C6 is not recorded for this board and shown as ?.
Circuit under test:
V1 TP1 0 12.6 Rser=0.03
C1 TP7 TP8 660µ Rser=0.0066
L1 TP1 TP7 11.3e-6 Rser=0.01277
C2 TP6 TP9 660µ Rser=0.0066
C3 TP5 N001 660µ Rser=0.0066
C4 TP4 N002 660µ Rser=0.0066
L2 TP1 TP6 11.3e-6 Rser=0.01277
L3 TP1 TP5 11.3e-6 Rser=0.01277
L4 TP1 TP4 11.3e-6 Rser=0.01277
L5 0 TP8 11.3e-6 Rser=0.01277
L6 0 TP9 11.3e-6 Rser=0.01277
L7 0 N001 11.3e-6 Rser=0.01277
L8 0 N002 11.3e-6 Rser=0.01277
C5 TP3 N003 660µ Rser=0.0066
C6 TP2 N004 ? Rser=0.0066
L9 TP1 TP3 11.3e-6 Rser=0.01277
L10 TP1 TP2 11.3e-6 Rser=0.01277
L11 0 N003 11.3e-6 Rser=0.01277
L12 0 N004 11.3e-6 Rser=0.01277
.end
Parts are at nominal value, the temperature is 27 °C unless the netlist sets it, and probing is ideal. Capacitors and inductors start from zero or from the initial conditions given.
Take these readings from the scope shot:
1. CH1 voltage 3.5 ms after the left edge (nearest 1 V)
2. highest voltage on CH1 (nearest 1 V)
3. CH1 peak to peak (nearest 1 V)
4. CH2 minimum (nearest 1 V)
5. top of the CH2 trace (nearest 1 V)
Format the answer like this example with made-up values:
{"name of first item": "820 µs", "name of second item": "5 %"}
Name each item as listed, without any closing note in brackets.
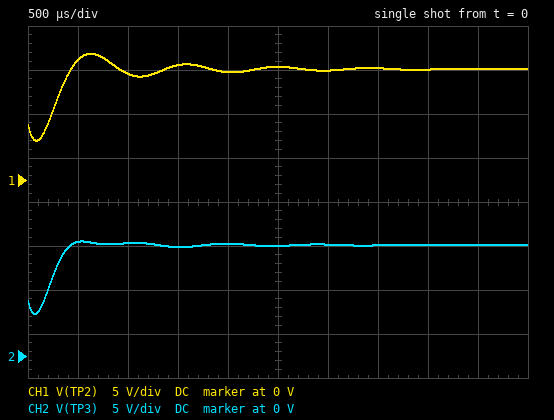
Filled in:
{"CH1 voltage 3.5 ms after the left edge": "13 V", "highest voltage on CH1": "14 V", "CH1 peak to peak": "10 V", "CH2 minimum": "5 V", "top of the CH2 trace": "13 V"}
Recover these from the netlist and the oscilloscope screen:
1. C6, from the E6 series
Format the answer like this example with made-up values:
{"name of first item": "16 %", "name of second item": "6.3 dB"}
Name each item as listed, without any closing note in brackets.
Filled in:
{"C6, from the E6 series": "1 mF"}
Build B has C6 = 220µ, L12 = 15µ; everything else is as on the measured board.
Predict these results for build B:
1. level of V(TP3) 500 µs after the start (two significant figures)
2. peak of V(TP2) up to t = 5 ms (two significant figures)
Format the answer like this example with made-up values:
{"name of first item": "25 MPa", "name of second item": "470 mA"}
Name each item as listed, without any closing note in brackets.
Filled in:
{"level of V(TP3) 500 µs after the start": "14 V", "peak of V(TP2) up to t = 5 ms": "16 V"}
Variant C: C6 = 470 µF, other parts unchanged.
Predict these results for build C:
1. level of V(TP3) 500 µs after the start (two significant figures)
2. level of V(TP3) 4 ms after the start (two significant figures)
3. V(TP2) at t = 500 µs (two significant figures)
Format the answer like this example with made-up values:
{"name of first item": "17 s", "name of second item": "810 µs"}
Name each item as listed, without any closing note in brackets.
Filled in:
{"level of V(TP3) 500 µs after the start": "14 V", "level of V(TP3) 4 ms after the start": "13 V", "V(TP2) at t = 500 µs": "12 V"}
